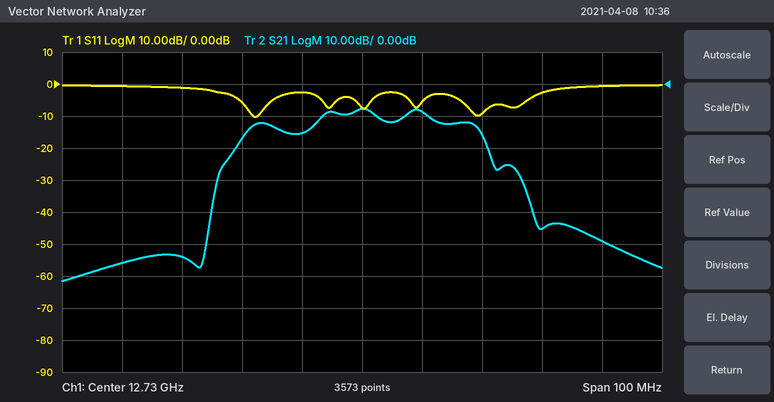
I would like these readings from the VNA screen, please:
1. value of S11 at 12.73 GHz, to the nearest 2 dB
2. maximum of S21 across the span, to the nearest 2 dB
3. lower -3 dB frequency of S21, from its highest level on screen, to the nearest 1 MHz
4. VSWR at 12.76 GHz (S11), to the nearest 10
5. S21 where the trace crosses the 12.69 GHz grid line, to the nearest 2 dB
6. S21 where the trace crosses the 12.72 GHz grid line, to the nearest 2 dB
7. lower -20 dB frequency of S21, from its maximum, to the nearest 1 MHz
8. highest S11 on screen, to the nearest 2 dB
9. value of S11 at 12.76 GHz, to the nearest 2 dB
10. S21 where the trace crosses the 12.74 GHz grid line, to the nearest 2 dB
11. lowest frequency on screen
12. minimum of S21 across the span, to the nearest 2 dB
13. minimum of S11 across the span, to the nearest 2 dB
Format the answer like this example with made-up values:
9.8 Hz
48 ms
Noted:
-8 dB
-8 dB
12.723 GHz
10
-56 dB
-16 dB
12.706 GHz
0 dB
-2 dB
-8 dB
12.68 GHz
-62 dB
-10 dB
